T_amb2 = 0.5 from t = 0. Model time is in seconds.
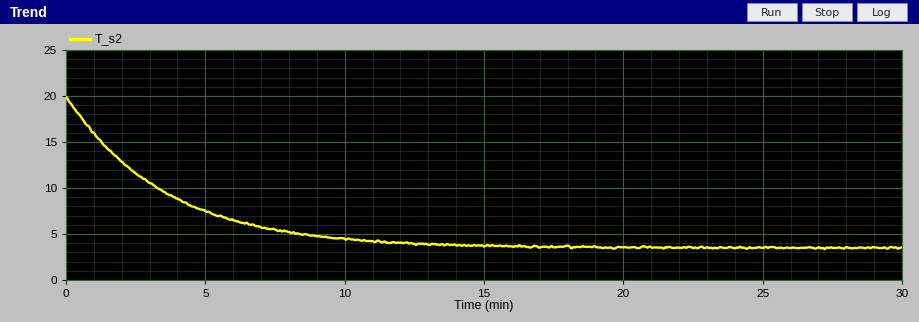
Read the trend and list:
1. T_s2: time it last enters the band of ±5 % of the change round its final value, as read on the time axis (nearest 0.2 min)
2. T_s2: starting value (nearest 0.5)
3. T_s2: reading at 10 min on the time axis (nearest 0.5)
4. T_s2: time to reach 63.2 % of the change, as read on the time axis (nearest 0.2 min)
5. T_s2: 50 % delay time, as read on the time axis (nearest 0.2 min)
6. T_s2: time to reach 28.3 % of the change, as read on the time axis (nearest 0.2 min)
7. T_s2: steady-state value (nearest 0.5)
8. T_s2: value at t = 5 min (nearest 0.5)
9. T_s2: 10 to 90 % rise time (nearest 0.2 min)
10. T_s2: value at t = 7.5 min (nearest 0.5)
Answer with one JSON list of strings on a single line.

["10.6 min", "20.0", "4.5", "3.6 min", "2.4 min", "1.2 min", "3.5", "7.5", "7.8 min", "5.5"]
